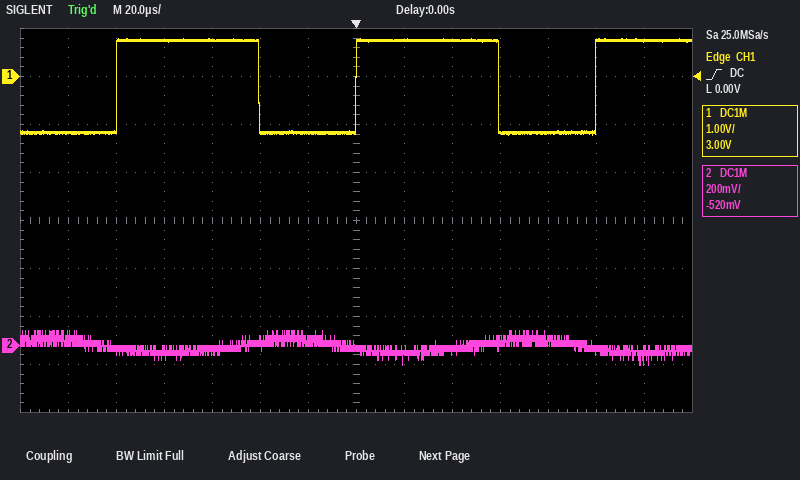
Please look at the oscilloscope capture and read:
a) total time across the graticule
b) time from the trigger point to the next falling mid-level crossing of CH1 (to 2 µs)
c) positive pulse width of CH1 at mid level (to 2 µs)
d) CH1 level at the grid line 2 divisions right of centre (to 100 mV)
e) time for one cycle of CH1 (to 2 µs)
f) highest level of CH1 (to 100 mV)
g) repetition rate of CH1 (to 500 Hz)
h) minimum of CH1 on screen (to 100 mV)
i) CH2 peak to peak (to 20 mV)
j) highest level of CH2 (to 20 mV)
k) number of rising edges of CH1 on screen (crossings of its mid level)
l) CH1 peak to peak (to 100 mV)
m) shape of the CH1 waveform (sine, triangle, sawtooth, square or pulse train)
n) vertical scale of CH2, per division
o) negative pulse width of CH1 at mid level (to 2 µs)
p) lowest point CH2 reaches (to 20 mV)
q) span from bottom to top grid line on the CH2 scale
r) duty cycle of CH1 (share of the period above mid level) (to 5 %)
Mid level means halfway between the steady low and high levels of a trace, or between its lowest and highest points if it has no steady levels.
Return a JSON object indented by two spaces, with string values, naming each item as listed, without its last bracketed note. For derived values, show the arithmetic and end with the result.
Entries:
{
  "total time across the graticule": "280 µs",
  "time from the trigger point to the next falling mid-level crossing of CH1": "60 µs",
  "positive pulse width of CH1 at mid level": "60 µs",
  "CH1 level at the grid line 2 divisions right of centre": "800 mV",
  "time for one cycle of CH1": "100 µs",
  "highest level of CH1": "800 mV",
  "repetition rate of CH1": "1 / 100 µs ≈ 10.0 kHz",
  "minimum of CH1 on screen": "-1.2 V",
  "CH2 peak to peak": "60 mV − (-80 mV) = 140 mV",
  "highest level of CH2": "60 mV",
  "number of rising edges of CH1 on screen": "3",
  "CH1 peak to peak": "800 mV − (-1.2 V) = 2.0 V",
  "shape of the CH1 waveform": "pulse train",
  "vertical scale of CH2, per division": "200 mV",
  "negative pulse width of CH1 at mid level": "40 µs",
  "lowest point CH2 reaches": "-80 mV",
  "span from bottom to top grid line on the CH2 scale": "1.6 V",
  "duty cycle of CH1 (share of the period above mid level)": "60 µs / 100 µs ≈ 60 %"
}
